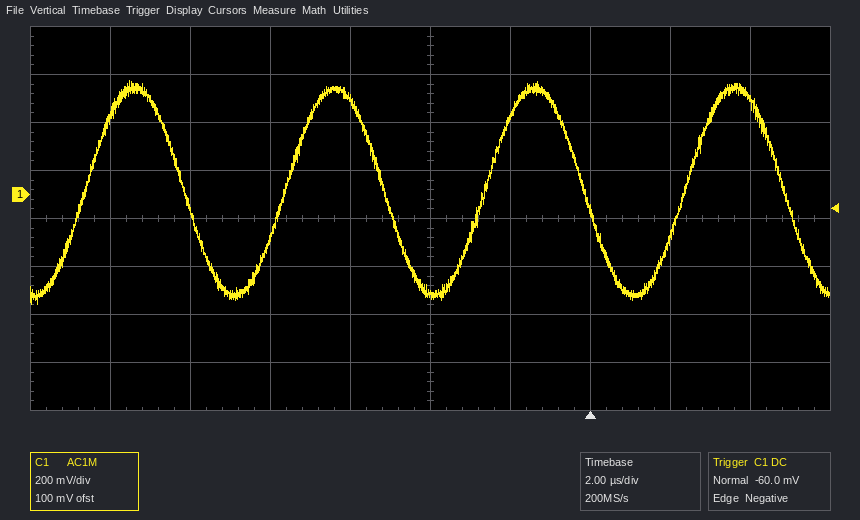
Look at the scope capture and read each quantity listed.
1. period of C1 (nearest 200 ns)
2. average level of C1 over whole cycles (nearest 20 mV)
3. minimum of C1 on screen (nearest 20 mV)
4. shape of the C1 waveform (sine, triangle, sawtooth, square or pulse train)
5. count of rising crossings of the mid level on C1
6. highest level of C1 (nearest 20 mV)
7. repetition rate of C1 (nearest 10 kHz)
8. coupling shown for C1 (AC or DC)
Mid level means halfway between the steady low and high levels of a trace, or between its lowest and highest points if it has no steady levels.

5.0 µs
20 mV
-460 mV
sine
4
480 mV
200 kHz
AC
